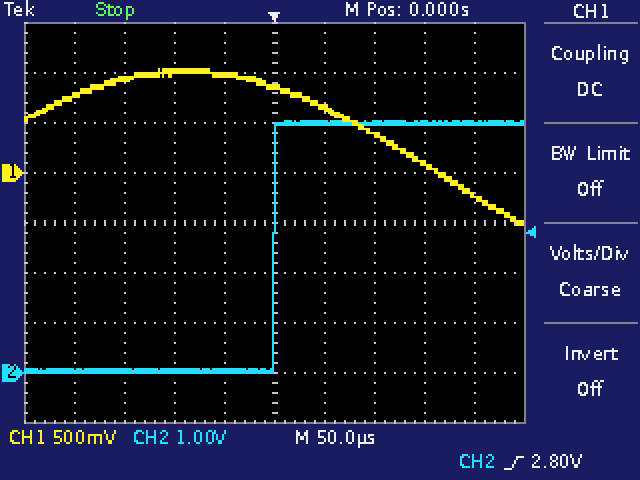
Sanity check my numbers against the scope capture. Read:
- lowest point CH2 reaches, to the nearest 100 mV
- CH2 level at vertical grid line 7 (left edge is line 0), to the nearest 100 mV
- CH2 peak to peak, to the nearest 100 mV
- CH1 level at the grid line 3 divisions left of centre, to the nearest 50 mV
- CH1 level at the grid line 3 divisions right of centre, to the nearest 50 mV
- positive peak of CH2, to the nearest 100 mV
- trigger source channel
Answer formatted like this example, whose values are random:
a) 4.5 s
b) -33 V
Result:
a) 0.0 V
b) 5.0 V
c) 5.0 V
d) 950 mV
e) 100 mV
f) 5.0 V
g) CH2
